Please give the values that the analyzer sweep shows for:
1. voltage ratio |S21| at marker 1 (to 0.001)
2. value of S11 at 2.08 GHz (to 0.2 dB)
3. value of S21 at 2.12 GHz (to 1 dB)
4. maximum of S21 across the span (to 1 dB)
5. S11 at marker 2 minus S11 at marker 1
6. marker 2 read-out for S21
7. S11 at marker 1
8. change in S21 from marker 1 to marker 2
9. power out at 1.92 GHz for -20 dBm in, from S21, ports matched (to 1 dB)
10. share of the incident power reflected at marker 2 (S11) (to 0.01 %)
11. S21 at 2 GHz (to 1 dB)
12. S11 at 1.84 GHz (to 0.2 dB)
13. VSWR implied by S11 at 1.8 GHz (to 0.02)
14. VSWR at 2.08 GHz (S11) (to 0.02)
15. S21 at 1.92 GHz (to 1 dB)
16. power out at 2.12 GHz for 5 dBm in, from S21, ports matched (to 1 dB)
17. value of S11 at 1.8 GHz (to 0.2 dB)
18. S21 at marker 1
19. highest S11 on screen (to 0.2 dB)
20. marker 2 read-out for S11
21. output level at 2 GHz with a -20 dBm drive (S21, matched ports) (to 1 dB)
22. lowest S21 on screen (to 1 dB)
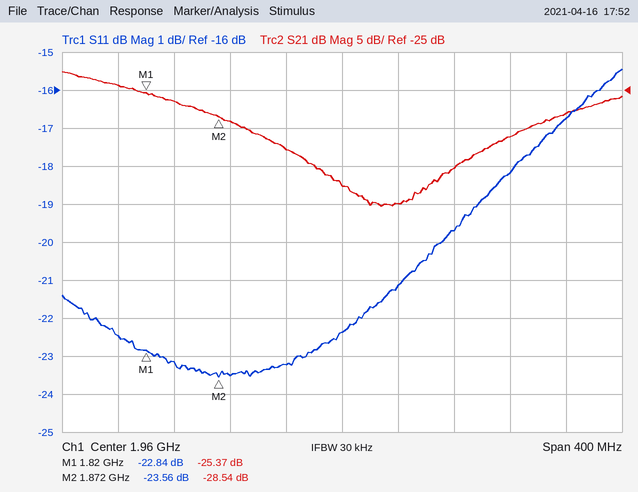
0.054
-18.2 dB
-28 dB
-23 dB
-0.72 dB
-28.54 dB
-22.84 dB
-3.17 dB
-53 dBm
0.44 %
-40 dB
-23.2 dB
1.16
1.28
-33 dB
-23 dBm
-22.4 dB
-25.37 dB
-15.4 dB
-23.56 dB
-60 dBm
-40 dB
